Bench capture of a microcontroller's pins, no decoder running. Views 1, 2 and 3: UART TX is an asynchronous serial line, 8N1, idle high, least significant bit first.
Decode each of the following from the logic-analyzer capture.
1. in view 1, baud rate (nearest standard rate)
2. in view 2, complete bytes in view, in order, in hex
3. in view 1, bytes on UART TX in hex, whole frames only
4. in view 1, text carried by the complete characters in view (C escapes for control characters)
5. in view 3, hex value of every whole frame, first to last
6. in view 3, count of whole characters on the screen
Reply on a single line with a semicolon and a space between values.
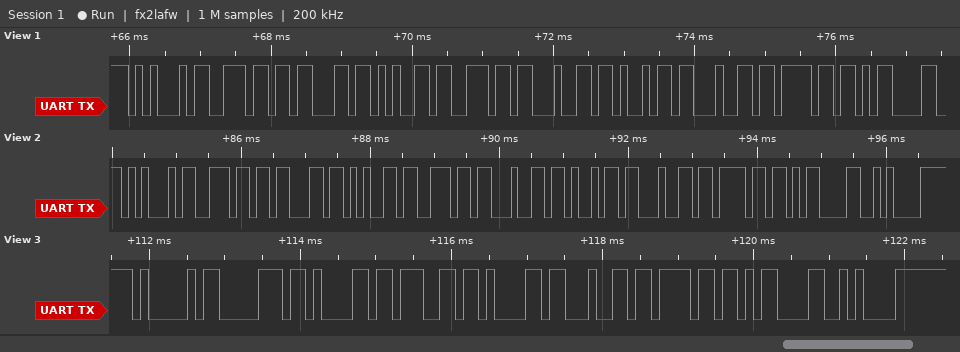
9600 baud; 0x45 0x6E 0x63 0x65 0x6E 0x64 0x69 0x64 0x6F 0x0D 0x0A; 45 6E 63 65 6E 64 69 64 6F 0D; "Encendido\r"; 41 70 61 67 61 64 6F 0D 0A; 9
